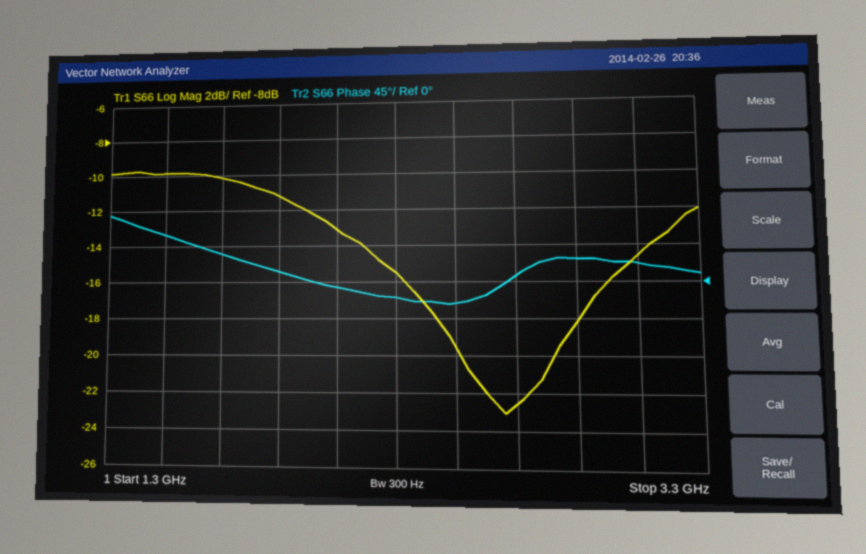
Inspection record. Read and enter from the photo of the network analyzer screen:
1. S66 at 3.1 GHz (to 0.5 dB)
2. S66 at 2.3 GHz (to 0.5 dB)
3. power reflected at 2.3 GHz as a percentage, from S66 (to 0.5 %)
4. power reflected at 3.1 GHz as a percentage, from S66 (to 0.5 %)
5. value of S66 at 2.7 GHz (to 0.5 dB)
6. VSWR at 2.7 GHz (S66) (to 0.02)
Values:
-14.5 dB
-15.5 dB
3.0 %
3.5 %
-22.5 dB
1.16
